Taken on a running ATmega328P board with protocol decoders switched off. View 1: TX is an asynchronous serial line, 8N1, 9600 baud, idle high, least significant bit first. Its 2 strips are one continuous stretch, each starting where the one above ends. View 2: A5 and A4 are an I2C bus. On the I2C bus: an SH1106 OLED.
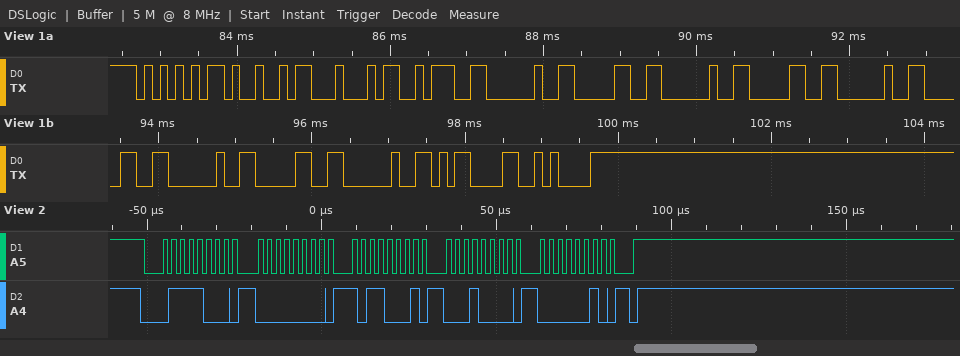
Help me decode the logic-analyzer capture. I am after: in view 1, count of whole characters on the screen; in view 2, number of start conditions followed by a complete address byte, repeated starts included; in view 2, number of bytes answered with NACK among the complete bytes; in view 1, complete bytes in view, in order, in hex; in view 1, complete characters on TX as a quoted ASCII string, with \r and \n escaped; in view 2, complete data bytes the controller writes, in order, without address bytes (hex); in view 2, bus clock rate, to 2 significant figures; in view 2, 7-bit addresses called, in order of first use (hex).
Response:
15
1
0
55 49 44 3A 20 30 20 30 20 30 20 30 20 0D 0A
"UID: 0 0 0 0 \r\n"
00 B1 10 02
400 kHz
0x3C
